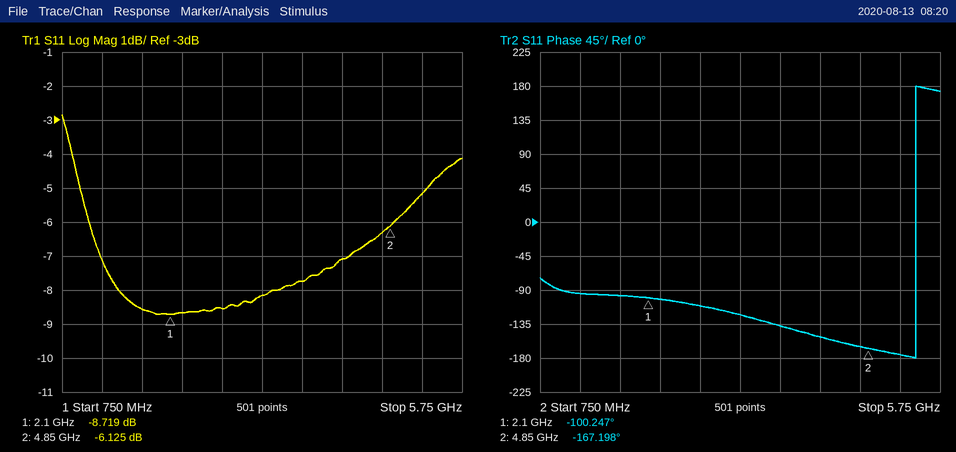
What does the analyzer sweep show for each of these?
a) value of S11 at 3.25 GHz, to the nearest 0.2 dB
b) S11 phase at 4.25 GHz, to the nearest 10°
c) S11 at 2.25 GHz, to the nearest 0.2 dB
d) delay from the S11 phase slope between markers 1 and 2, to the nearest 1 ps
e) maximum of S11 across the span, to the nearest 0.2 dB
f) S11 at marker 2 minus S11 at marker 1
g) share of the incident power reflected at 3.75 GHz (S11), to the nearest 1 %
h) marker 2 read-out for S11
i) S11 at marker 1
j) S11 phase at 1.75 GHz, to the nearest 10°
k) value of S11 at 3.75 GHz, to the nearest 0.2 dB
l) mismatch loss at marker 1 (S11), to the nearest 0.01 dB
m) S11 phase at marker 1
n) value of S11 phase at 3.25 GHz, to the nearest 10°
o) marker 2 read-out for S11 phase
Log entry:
-8.2 dB
-150°
-8.6 dB
68 ps
-2.8 dB
2.594 dB
17 %
-6.125 dB
-8.719 dB
-100°
-7.8 dB
0.63 dB
-100.247°
-120°
-167.198°
